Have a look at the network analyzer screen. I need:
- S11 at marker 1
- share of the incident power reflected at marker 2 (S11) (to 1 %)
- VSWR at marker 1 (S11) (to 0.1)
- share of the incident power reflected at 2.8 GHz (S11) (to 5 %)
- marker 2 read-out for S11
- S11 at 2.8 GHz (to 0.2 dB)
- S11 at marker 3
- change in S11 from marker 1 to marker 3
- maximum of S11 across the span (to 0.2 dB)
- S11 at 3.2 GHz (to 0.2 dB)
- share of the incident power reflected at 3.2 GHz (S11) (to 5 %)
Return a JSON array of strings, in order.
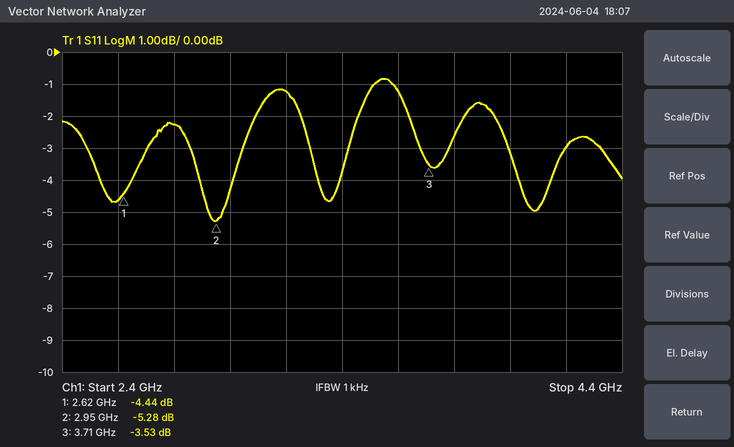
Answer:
["-4.44 dB", "30 %", "4.0", "60 %", "-5.28 dB", "-2.2 dB", "-3.53 dB", "0.91 dB", "-0.8 dB", "-1.2 dB", "75 %"]
